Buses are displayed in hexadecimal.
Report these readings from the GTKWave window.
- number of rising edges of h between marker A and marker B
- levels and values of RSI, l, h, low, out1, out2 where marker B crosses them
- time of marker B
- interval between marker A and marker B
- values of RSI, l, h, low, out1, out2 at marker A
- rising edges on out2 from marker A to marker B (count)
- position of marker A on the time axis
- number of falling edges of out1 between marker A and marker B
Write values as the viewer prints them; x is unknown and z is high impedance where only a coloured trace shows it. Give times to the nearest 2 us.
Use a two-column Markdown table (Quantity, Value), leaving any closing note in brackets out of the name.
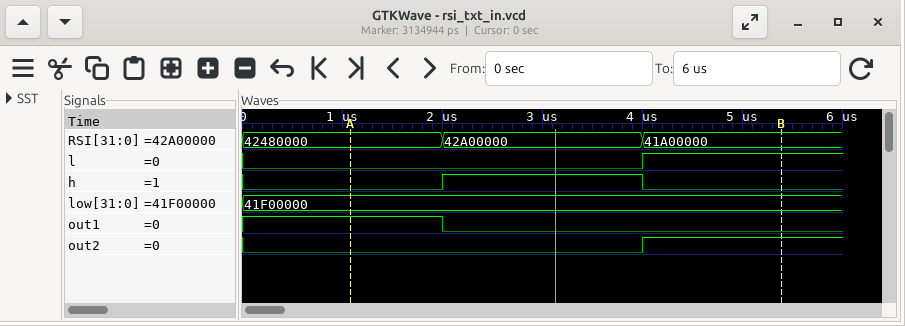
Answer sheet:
| Quantity | Value |
|---|---|
| number of rising edges of h between marker A and marker B | 1 |
| levels and values of RSI, l, h, low, out1, out2 where marker B crosses them | RSI=41A00000, l=1, h=0, low=41F00000, out1=0, out2=1 |
| time of marker B | 6 us |
| interval between marker A and marker B | 4 us |
| values of RSI, l, h, low, out1, out2 at marker A | RSI=42480000, l=0, h=0, low=41F00000, out1=1, out2=0 |
| rising edges on out2 from marker A to marker B | 1 |
| position of marker A on the time axis | 2 us |
| number of falling edges of out1 between marker A and marker B | 1 |
